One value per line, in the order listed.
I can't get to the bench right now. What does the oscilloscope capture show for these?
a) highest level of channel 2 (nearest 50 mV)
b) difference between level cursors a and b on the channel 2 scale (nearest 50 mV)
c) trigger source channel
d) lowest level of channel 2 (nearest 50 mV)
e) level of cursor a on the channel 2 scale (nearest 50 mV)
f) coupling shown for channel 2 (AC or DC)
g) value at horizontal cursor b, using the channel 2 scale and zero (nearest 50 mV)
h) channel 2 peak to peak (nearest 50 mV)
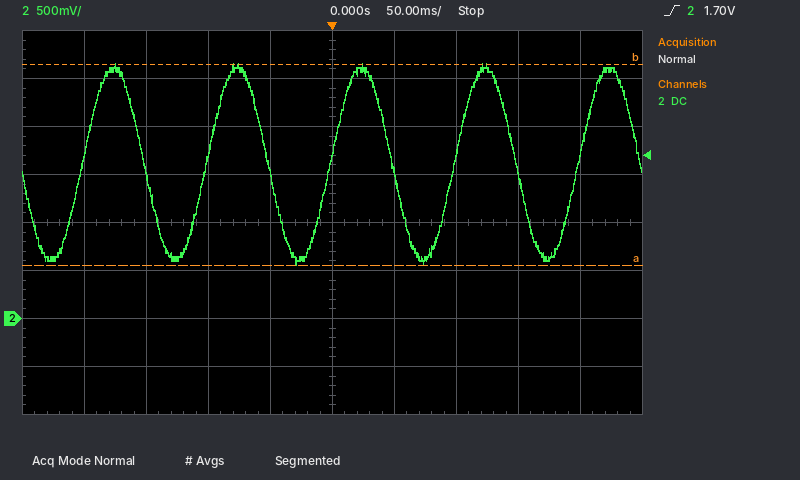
2.65 V
2.10 V
channel 2
550 mV
550 mV
DC
2.65 V
2.10 V
